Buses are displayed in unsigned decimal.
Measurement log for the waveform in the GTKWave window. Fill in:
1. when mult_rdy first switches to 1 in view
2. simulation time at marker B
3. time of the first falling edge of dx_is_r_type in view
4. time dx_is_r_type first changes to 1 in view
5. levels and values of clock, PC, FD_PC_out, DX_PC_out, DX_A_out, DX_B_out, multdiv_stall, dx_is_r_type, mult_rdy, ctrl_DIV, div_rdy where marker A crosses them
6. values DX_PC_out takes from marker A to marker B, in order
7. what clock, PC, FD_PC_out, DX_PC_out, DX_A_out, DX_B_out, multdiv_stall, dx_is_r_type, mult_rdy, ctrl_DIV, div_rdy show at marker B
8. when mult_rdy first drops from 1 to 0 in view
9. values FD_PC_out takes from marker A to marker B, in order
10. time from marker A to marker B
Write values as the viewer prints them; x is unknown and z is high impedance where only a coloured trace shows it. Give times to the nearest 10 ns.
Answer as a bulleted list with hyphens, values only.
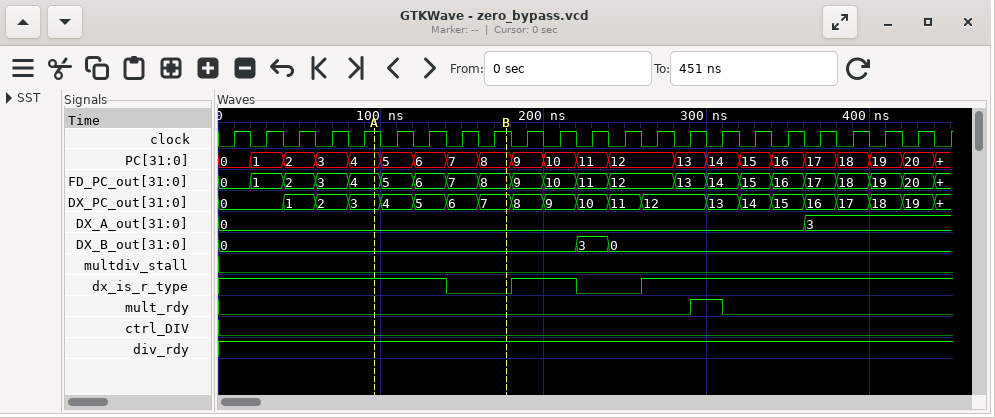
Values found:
- 290 ns
- 180 ns
- 140 ns
- 180 ns
- clock=1, PC=4, FD_PC_out=4, DX_PC_out=3, DX_A_out=0, DX_B_out=0, multdiv_stall=0, dx_is_r_type=1, mult_rdy=0, ctrl_DIV=0, div_rdy=1
- 3, 4, 5, 6, 7
- clock=1, PC=8, FD_PC_out=8, DX_PC_out=7, DX_A_out=0, DX_B_out=0, multdiv_stall=0, dx_is_r_type=0, mult_rdy=0, ctrl_DIV=0, div_rdy=1
- 310 ns
- 4, 5, 6, 7, 8
- 80 ns
